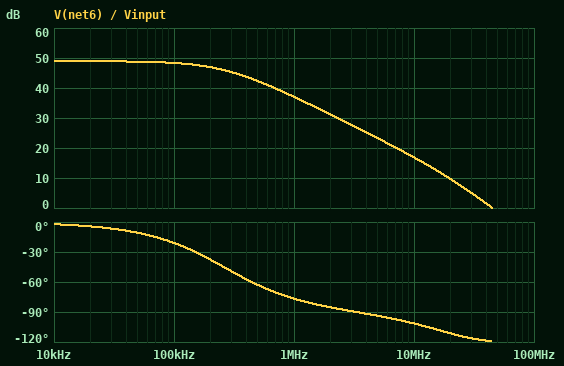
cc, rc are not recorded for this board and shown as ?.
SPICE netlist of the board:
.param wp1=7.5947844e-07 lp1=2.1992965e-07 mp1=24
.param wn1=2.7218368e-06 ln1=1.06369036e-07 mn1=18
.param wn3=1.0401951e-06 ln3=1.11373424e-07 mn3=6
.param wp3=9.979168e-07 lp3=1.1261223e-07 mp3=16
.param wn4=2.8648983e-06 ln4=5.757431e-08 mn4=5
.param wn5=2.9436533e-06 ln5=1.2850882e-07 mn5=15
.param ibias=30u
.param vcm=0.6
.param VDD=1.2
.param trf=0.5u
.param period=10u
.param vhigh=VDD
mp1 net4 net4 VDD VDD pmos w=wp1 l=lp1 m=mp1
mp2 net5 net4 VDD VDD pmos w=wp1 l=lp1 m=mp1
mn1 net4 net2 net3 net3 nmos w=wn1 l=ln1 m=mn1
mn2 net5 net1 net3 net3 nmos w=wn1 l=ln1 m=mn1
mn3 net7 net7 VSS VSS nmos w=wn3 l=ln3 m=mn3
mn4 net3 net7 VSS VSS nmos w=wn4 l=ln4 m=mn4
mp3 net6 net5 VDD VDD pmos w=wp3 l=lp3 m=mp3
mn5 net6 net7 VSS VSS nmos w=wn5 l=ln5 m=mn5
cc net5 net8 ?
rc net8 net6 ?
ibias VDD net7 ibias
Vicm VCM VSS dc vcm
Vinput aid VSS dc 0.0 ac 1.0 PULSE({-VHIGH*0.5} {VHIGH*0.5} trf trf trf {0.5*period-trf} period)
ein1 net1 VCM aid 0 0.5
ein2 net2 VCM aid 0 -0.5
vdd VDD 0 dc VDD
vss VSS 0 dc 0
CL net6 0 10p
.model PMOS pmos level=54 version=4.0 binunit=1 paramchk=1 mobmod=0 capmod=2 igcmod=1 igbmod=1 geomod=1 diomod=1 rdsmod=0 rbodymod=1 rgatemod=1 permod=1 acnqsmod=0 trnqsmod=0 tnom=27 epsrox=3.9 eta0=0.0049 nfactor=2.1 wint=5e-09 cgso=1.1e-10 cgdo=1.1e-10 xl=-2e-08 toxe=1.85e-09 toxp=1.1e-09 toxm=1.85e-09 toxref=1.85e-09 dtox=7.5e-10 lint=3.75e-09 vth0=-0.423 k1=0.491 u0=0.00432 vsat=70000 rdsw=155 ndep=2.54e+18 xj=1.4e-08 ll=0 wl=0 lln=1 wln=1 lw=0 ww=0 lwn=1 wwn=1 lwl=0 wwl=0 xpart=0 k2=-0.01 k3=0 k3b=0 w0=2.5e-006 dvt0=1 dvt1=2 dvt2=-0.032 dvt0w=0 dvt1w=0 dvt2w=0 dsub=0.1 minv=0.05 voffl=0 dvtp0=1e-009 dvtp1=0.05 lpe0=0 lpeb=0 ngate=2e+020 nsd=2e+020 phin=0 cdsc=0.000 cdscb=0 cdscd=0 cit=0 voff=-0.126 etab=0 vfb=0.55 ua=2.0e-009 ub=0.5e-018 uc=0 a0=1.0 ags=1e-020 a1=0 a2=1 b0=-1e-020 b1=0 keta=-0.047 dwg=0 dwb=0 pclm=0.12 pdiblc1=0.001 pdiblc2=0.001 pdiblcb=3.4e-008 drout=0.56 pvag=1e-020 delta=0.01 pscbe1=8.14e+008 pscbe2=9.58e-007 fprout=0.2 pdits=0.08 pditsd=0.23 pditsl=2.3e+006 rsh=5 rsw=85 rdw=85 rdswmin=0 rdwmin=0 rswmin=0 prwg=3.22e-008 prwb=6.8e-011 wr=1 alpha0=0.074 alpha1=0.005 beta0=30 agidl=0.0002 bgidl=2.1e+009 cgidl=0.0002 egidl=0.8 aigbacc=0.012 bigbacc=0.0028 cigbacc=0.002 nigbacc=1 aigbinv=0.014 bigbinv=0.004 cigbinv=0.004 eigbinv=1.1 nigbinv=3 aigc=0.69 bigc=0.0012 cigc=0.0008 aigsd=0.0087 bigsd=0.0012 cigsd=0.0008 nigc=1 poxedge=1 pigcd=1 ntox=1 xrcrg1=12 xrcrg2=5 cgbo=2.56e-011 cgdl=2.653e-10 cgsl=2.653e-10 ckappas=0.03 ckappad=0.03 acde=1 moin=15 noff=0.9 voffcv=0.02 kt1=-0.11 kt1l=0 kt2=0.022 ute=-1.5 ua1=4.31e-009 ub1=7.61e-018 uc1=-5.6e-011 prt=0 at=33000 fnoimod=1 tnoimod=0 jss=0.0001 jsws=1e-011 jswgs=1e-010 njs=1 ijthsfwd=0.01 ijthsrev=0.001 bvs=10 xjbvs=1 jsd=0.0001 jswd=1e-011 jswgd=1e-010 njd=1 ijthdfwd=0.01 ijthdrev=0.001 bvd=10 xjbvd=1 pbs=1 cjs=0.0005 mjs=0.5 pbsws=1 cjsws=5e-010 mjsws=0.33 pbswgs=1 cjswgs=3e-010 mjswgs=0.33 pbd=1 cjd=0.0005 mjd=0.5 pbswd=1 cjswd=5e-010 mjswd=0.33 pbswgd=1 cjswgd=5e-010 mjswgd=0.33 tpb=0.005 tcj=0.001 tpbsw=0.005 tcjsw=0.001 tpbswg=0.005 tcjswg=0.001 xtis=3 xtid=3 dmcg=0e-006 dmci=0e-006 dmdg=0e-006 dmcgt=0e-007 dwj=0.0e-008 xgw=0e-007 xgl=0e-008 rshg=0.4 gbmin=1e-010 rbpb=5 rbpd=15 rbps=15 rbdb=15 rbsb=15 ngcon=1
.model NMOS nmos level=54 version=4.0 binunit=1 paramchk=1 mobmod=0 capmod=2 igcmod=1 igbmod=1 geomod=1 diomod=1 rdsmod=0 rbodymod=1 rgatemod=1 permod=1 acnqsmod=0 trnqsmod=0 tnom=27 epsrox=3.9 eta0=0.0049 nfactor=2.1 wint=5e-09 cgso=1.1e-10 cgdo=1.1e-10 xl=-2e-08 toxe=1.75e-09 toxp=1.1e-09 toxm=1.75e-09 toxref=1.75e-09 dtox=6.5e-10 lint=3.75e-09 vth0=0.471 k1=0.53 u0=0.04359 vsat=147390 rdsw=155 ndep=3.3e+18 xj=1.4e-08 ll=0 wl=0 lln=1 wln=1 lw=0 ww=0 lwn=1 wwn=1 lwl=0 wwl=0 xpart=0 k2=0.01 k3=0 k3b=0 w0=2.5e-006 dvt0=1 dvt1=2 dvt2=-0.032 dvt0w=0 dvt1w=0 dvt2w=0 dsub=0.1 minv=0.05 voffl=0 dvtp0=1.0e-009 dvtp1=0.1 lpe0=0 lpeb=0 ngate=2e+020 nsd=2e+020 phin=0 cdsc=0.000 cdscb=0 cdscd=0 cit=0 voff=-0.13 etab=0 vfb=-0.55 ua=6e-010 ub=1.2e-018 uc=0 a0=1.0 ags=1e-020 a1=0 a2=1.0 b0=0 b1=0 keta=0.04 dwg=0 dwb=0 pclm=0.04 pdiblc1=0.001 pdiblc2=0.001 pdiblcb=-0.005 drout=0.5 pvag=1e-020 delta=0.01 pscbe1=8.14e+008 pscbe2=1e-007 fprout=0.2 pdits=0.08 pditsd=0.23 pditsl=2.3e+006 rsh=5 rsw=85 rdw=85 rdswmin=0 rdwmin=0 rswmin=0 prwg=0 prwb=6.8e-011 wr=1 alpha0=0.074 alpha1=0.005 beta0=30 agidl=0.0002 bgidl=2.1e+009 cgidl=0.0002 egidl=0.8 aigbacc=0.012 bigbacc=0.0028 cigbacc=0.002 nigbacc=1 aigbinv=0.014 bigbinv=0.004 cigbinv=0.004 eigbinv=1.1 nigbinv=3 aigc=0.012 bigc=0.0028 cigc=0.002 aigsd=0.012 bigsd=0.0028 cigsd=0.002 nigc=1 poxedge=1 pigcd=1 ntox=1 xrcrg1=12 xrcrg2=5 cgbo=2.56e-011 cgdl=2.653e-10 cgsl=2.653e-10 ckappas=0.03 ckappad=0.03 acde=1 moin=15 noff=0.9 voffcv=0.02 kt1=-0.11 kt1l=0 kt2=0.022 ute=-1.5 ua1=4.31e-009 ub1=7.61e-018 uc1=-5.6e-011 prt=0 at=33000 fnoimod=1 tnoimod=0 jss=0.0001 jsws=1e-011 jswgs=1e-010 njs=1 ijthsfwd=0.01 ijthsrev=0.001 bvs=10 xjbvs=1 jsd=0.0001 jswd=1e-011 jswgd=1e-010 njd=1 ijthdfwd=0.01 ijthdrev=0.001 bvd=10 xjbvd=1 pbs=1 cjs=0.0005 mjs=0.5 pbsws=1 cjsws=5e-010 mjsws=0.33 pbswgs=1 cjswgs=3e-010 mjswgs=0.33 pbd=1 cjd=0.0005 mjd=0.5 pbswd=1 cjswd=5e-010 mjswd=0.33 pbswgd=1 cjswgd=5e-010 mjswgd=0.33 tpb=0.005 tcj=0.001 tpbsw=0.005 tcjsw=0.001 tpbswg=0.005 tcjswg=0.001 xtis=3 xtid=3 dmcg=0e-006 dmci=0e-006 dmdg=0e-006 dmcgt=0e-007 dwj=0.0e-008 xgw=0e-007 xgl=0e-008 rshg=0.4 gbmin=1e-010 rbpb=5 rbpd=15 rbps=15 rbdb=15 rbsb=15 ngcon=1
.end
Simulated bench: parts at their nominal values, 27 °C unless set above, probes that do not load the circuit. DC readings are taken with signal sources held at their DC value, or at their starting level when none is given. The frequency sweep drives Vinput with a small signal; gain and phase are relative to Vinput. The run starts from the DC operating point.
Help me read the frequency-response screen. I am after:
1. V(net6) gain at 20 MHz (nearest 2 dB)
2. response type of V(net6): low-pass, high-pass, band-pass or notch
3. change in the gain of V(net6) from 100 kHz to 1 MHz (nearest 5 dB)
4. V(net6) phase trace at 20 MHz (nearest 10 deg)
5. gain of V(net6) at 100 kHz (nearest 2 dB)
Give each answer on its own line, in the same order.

10 dB
low-pass
-10 dB
-110 deg
48 dB
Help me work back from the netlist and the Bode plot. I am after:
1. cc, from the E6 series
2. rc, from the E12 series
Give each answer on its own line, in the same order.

3.3 pF
1.5 kΩ
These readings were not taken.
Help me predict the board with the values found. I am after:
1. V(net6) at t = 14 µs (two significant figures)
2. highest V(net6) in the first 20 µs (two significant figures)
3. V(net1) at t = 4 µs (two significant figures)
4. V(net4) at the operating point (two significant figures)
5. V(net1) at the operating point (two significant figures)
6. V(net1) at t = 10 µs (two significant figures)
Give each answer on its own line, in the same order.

1.2 V
1.2 V
900 mV
560 mV
600 mV
300 mV
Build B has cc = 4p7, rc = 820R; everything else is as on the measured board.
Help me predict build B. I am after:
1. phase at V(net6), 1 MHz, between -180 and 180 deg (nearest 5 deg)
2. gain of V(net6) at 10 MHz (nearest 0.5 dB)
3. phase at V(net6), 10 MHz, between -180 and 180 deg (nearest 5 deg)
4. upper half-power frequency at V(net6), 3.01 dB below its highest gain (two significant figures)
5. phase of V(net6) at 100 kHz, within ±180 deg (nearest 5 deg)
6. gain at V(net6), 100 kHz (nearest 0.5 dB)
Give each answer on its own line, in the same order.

-80 deg
14.0 dB
-110 deg
190 kHz
-30 deg
48.0 dB
